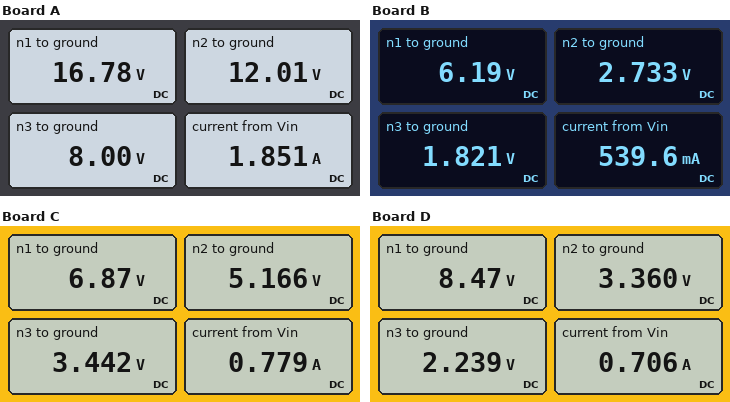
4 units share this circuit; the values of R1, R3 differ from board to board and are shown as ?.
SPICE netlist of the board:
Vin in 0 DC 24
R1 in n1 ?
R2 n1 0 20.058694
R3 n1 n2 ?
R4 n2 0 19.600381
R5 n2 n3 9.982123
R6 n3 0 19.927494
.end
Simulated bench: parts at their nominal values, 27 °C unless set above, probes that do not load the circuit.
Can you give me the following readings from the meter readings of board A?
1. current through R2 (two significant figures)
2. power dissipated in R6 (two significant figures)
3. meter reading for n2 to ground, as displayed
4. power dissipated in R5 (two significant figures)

840 mA
3.2 W
12.01 V
1.6 W
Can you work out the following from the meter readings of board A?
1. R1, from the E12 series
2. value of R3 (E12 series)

3.9 Ω
4.7 Ω
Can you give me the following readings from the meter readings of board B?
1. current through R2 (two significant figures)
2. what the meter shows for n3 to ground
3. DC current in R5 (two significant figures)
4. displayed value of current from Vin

310 mA
1.821 V
91 mA
539.6 mA
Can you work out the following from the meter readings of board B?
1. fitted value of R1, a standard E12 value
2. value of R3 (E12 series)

33 Ω
15 Ω
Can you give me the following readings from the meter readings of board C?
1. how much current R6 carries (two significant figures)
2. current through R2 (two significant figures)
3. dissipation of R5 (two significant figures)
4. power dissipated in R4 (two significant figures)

170 mA
340 mA
300 mW
1.4 W
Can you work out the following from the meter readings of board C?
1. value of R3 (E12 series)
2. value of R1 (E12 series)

3.9 Ω
22 Ω
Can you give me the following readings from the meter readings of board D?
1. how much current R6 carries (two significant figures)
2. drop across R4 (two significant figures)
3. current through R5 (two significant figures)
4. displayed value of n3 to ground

110 mA
3.4 V
110 mA
2.239 V
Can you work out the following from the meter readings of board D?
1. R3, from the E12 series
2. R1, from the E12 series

18 Ω
22 Ω
